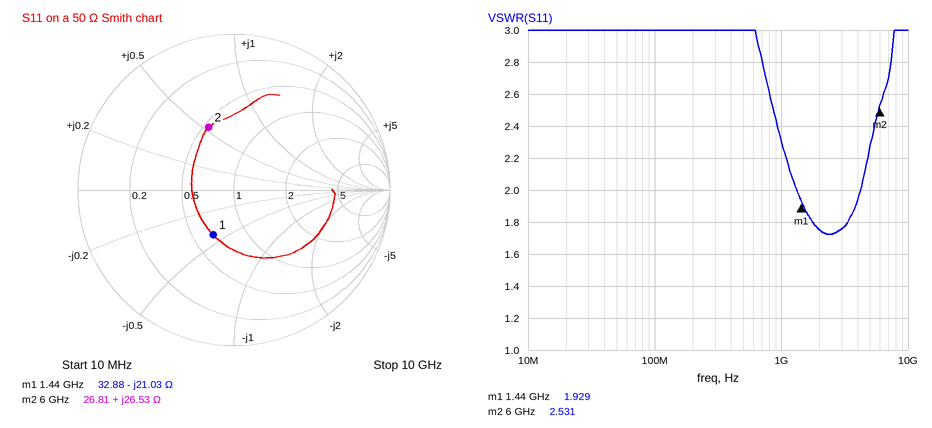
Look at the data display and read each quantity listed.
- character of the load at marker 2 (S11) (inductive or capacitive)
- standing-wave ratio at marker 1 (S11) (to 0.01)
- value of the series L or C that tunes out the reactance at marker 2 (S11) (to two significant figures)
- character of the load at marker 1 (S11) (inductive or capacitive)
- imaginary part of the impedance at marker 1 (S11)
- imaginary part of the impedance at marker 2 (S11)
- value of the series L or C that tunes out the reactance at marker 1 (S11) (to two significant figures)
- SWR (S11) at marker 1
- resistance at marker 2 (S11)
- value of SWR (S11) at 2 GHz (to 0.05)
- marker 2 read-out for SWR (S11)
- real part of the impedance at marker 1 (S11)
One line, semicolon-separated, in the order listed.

inductive; 1.93; 1.00 pF; capacitive; -21.03 Ω; +26.53 Ω; 2.3 nH; 1.929; 26.81 Ω; 1.75; 2.531; 32.88 Ω
